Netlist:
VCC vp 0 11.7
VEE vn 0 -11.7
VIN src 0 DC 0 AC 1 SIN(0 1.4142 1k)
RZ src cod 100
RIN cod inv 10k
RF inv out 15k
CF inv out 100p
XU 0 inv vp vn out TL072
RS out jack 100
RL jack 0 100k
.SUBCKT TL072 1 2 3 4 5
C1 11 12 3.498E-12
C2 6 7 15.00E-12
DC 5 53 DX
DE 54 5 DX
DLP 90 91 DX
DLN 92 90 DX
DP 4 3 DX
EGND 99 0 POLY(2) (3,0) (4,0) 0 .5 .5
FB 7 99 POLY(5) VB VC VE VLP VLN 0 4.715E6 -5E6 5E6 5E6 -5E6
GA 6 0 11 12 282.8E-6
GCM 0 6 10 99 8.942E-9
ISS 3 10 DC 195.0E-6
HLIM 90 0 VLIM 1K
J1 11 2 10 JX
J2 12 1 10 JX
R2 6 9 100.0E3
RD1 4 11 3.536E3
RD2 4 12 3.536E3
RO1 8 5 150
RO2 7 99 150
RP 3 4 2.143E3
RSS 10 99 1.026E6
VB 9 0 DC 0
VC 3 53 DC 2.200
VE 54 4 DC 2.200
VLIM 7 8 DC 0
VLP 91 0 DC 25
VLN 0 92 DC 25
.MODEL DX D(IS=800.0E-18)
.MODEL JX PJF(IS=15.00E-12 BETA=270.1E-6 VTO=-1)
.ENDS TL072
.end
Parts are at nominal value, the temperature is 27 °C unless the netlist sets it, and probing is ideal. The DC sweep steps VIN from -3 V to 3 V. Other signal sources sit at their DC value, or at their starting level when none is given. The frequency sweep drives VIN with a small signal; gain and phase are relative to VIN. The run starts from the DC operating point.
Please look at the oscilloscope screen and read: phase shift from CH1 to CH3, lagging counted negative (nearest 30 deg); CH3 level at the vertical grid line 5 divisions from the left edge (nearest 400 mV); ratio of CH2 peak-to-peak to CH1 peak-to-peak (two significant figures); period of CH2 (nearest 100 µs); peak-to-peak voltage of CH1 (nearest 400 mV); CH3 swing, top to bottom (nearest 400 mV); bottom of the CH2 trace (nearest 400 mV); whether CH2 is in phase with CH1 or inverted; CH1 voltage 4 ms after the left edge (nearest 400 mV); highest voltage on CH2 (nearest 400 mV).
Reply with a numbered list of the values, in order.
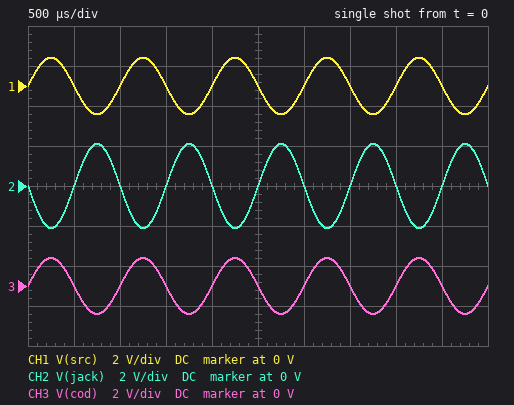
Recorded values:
1. 0 deg
2. 0 V
3. 1.5
4. 1.0 ms
5. 2.8 V
6. 2.8 V
7. -2.0 V
8. inverted
9. 0 V
10. 2.0 V
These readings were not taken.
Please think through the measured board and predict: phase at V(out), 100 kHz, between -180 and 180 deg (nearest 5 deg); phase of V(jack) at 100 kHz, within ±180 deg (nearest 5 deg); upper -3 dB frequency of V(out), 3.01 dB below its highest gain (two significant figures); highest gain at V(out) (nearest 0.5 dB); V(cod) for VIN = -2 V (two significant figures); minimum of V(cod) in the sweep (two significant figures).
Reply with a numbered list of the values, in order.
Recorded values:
1. 135 deg
2. 135 deg
3. 100 kHz
4. 3.5 dB
5. -2.0 V
6. -3.0 V
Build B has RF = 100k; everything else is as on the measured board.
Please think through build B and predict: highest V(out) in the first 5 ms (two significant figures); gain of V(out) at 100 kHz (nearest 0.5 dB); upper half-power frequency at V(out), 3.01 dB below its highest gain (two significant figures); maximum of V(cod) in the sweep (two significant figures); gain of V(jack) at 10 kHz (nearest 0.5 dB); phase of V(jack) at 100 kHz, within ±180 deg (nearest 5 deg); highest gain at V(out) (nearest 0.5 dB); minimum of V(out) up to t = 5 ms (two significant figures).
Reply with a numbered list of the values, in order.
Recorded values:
1. 10 V
2. 3.5 dB
3. 15 kHz
4. 3.0 V
5. 18.5 dB
6. 95 deg
7. 20.0 dB
8. -10 V
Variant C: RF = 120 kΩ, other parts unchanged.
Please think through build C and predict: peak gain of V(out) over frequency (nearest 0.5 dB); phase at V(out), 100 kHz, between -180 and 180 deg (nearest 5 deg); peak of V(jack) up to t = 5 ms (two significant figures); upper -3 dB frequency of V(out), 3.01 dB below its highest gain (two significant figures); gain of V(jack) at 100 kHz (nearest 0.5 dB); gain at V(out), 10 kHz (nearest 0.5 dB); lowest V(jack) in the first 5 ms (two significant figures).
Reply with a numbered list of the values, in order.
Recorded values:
1. 21.5 dB
2. 95 deg
3. 10 V
4. 13 kHz
5. 3.5 dB
6. 19.5 dB
7. -10 V
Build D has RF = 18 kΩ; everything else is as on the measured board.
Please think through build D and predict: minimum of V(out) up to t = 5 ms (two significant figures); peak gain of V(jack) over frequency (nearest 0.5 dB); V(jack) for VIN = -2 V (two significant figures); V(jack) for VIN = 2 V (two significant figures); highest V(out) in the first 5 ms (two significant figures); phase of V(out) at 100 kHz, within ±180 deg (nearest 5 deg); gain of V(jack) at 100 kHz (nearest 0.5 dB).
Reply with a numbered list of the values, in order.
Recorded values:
1. -2.5 V
2. 5.0 dB
3. 3.6 V
4. -3.6 V
5. 2.5 V
6. 130 deg
7. 1.0 dB
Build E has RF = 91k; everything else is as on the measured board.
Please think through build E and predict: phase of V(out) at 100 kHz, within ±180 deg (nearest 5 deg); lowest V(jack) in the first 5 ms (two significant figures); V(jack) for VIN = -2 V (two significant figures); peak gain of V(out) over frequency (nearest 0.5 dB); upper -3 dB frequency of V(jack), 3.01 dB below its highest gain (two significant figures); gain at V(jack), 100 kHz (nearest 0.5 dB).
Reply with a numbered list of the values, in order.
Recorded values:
1. 100 deg
2. -10 V
3. 10 V
4. 19.0 dB
5. 17 kHz
6. 3.5 dB
